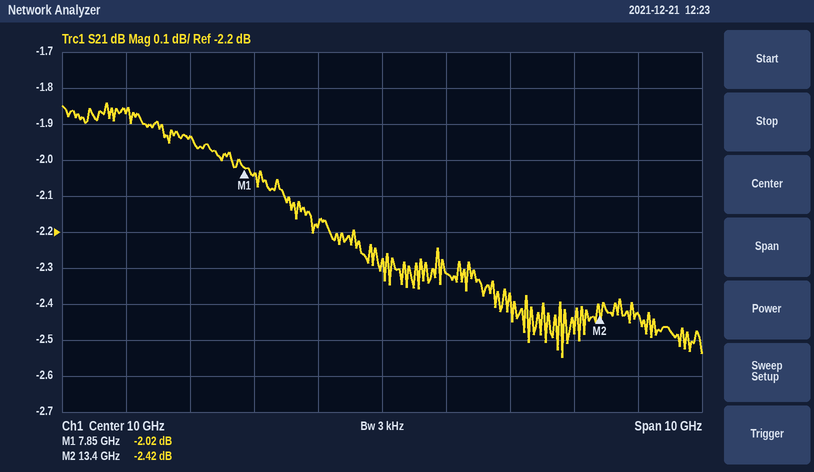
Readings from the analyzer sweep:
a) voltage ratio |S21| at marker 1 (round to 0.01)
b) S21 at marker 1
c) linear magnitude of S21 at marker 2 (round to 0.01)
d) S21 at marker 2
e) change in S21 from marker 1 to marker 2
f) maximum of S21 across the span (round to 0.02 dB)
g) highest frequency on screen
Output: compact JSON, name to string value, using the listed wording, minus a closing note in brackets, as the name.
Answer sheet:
{"voltage ratio |S21| at marker 1": "0.79", "S21 at marker 1": "-2.02 dB", "linear magnitude of S21 at marker 2": "0.76", "S21 at marker 2": "-2.42 dB", "change in S21 from marker 1 to marker 2": "-0.40 dB", "maximum of S21 across the span": "-1.84 dB", "highest frequency on screen": "15 GHz"}
